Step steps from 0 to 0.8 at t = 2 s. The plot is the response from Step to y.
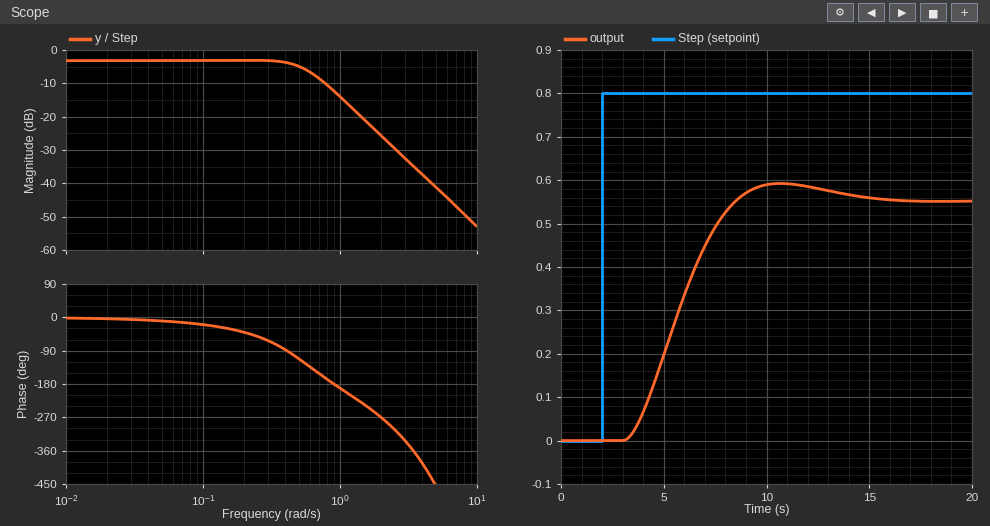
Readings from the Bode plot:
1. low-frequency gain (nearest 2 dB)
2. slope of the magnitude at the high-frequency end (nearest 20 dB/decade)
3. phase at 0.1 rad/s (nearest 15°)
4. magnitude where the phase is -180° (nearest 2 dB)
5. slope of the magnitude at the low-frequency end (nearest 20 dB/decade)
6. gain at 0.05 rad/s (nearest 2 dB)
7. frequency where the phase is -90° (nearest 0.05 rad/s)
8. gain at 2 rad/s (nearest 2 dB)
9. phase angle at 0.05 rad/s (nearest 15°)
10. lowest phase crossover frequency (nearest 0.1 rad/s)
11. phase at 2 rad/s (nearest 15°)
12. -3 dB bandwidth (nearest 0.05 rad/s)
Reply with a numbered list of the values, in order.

1. -4 dB
2. -40 dB/decade
3. -15°
4. -12 dB
5. 0 dB/decade
6. -4 dB
7. 0.40 rad/s
8. -26 dB
9. -15°
10. 0.9 rad/s
11. -270°
12. 0.60 rad/s
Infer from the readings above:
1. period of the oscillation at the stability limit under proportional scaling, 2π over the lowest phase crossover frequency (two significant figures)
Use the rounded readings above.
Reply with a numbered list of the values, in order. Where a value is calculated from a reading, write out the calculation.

1. 2π / 0.9 = 7.0 s
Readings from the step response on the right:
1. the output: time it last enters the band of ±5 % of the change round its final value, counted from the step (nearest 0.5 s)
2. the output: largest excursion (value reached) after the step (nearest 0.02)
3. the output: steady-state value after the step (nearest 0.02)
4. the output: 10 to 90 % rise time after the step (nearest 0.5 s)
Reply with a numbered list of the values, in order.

1. 10.5 s
2. 0.60
3. 0.56
4. 3.5 s
